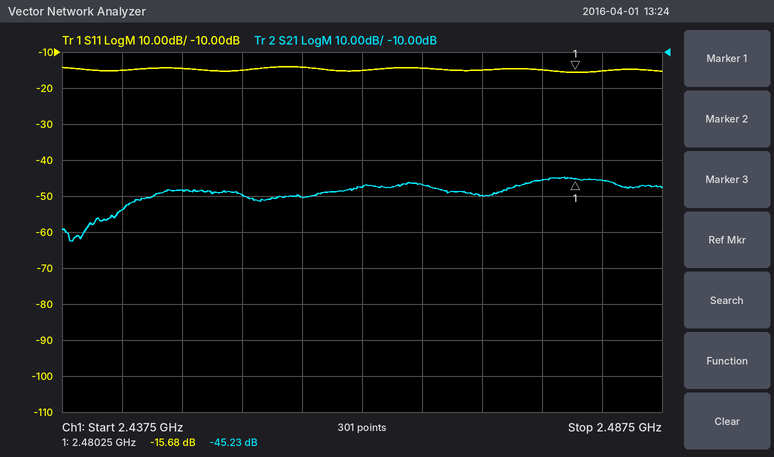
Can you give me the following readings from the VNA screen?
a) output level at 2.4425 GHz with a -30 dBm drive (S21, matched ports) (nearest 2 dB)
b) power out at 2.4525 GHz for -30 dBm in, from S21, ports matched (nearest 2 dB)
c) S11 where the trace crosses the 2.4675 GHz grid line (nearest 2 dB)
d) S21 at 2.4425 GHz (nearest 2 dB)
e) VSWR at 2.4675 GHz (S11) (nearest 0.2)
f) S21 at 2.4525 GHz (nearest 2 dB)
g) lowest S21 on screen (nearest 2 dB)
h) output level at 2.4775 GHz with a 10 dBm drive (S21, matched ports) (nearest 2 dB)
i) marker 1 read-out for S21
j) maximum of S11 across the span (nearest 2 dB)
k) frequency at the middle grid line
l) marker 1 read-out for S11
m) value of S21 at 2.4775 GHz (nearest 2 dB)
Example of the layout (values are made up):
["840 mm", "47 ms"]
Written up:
["-84 dBm", "-80 dBm", "-14 dB", "-54 dB", "1.4", "-50 dB", "-62 dB", "-36 dBm", "-45.23 dB", "-14 dB", "2.4625 GHz", "-15.68 dB", "-46 dB"]
